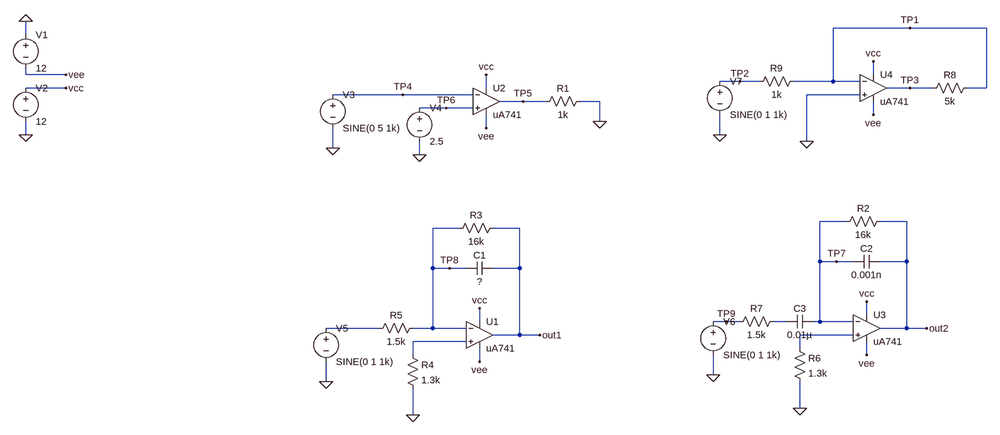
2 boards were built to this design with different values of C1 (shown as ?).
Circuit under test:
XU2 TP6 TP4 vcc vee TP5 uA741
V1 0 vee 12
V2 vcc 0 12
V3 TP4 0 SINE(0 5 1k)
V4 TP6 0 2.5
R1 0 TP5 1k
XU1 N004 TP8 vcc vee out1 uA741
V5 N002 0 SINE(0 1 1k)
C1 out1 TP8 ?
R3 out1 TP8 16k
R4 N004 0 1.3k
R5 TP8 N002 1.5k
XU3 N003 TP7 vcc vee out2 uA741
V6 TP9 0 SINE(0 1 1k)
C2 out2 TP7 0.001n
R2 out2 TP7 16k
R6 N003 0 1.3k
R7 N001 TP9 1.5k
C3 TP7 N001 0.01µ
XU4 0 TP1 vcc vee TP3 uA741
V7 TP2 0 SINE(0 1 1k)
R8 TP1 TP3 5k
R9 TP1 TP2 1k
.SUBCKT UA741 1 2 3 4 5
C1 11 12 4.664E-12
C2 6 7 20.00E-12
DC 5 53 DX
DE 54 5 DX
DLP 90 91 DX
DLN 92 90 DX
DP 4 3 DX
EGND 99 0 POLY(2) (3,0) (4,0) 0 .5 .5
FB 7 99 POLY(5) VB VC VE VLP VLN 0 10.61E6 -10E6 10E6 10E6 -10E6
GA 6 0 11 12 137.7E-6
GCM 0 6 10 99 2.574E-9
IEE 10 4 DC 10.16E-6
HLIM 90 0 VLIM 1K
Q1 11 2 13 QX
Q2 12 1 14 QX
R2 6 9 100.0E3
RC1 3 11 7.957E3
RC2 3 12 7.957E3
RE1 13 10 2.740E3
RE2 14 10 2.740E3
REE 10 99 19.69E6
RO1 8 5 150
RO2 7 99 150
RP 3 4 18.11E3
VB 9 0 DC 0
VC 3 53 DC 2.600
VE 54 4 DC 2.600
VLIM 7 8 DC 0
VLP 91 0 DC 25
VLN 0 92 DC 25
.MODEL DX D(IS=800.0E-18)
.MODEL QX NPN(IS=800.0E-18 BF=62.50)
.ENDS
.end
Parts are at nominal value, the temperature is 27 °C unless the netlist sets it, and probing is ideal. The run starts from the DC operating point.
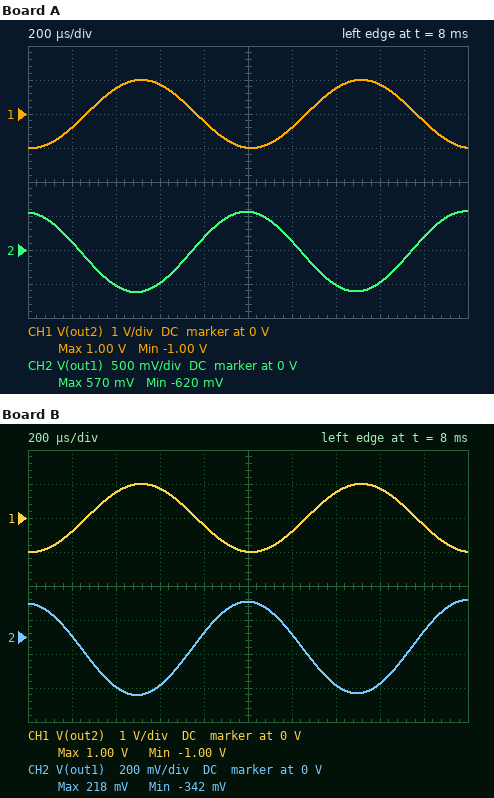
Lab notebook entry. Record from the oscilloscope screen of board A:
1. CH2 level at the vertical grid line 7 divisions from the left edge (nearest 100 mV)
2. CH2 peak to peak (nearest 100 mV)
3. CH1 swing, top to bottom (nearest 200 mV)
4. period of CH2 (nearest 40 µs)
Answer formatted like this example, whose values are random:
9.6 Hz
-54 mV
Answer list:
-500 mV
1.2 V
2.0 V
1.00 ms
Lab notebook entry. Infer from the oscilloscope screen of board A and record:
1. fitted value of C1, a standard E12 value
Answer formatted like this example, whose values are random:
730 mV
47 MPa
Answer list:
180 nF
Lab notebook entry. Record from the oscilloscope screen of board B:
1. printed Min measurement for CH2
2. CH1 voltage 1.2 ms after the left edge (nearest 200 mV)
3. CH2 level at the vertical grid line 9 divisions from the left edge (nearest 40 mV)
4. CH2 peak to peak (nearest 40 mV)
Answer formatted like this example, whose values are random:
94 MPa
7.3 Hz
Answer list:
-342 mV
-400 mV
40 mV
560 mV
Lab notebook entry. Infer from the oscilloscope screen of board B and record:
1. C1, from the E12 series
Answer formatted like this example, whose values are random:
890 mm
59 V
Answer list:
390 nF
